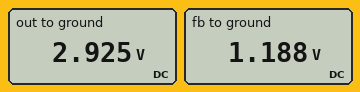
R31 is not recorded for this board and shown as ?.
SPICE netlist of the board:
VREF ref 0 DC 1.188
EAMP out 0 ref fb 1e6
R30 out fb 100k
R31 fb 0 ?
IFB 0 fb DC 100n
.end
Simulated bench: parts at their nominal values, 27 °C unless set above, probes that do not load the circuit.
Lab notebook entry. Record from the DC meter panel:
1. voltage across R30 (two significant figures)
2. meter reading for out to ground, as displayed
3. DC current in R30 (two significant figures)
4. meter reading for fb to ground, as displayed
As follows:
1.7 V
2.925 V
17 µA
1.188 V
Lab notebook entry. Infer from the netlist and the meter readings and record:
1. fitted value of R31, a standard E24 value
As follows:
68 kΩ
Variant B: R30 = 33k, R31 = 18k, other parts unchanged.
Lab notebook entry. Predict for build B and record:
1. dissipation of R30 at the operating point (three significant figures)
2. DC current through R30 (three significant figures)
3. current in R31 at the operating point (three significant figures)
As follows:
143 µW
65.9 µA
66.0 µA
